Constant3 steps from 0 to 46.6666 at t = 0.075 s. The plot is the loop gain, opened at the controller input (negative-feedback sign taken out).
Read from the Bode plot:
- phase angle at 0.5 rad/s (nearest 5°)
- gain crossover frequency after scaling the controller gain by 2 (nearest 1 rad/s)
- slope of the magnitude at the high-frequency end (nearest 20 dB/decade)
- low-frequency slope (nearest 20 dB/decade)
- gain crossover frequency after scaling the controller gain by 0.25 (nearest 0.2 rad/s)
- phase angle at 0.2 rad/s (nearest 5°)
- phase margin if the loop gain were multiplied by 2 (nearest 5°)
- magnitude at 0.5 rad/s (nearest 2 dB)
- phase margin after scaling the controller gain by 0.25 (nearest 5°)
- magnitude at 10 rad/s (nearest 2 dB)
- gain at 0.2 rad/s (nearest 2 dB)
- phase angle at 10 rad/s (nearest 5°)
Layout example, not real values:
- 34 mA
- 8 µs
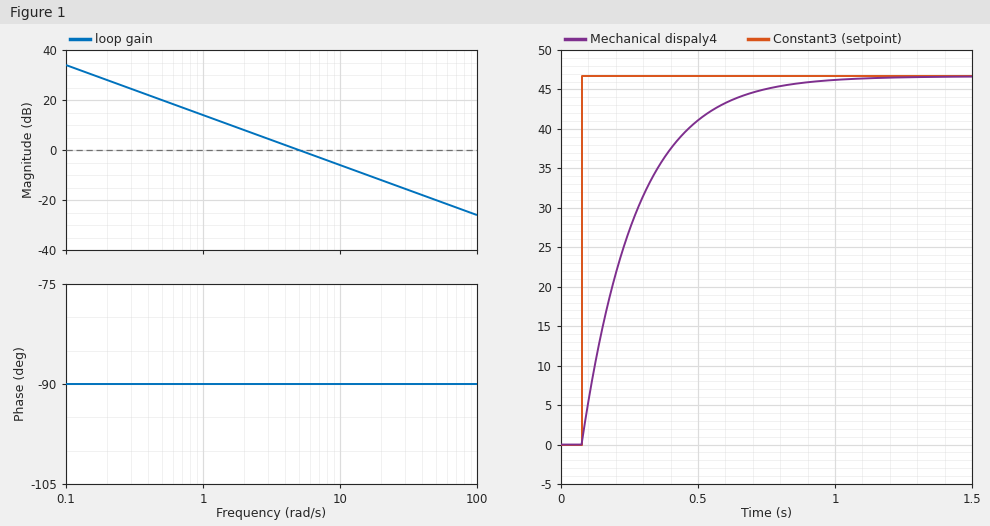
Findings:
- -90°
- 10 rad/s
- -20 dB/decade
- -20 dB/decade
- 1.2 rad/s
- -90°
- 90°
- 20 dB
- 90°
- -6 dB
- 28 dB
- -90°
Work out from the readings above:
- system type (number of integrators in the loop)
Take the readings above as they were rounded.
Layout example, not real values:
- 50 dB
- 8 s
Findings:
- 1
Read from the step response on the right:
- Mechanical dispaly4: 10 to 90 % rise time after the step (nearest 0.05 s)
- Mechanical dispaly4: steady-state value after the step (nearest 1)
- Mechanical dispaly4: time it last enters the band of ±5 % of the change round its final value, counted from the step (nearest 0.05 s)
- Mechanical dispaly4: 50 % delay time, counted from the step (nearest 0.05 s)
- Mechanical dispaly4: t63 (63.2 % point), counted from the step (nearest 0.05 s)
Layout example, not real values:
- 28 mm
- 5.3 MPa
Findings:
- 0.45 s
- 47
- 0.60 s
- 0.15 s
- 0.20 s
